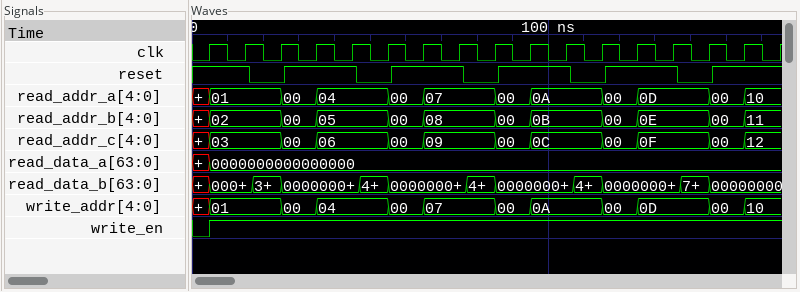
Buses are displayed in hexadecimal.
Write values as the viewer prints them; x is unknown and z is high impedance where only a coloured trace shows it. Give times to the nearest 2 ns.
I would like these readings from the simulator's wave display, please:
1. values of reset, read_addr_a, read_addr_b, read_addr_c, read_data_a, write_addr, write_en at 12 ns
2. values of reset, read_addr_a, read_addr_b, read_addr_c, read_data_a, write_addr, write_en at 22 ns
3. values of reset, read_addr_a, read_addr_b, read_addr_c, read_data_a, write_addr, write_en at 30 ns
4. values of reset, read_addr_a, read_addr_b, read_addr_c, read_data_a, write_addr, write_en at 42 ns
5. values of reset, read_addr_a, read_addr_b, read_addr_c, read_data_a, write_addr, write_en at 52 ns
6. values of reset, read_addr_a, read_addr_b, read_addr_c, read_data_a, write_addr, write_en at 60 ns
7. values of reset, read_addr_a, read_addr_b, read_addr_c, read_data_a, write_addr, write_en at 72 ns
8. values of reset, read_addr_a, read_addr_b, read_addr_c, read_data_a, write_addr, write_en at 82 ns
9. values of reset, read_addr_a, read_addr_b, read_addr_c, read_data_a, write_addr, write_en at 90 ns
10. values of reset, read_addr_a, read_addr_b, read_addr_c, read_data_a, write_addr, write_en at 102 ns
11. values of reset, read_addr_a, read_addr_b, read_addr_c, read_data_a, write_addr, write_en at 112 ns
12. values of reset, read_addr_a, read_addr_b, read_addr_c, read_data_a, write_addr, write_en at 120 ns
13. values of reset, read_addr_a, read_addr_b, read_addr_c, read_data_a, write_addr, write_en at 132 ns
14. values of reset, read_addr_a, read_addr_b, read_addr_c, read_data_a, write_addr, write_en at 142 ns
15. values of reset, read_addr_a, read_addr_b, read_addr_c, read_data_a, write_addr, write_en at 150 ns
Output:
reset=1, read_addr_a=01, read_addr_b=02, read_addr_c=03, read_data_a=0000000000000000, write_addr=01, write_en=1
reset=0, read_addr_a=01, read_addr_b=02, read_addr_c=03, read_data_a=0000000000000000, write_addr=01, write_en=1
reset=1, read_addr_a=00, read_addr_b=00, read_addr_c=00, read_data_a=0000000000000000, write_addr=00, write_en=1
reset=1, read_addr_a=04, read_addr_b=05, read_addr_c=06, read_data_a=0000000000000000, write_addr=04, write_en=1
reset=0, read_addr_a=04, read_addr_b=05, read_addr_c=06, read_data_a=0000000000000000, write_addr=04, write_en=1
reset=1, read_addr_a=00, read_addr_b=00, read_addr_c=00, read_data_a=0000000000000000, write_addr=00, write_en=1
reset=1, read_addr_a=07, read_addr_b=08, read_addr_c=09, read_data_a=0000000000000000, write_addr=07, write_en=1
reset=0, read_addr_a=07, read_addr_b=08, read_addr_c=09, read_data_a=0000000000000000, write_addr=07, write_en=1
reset=1, read_addr_a=00, read_addr_b=00, read_addr_c=00, read_data_a=0000000000000000, write_addr=00, write_en=1
reset=1, read_addr_a=0A, read_addr_b=0B, read_addr_c=0C, read_data_a=0000000000000000, write_addr=0A, write_en=1
reset=0, read_addr_a=0A, read_addr_b=0B, read_addr_c=0C, read_data_a=0000000000000000, write_addr=0A, write_en=1
reset=1, read_addr_a=00, read_addr_b=00, read_addr_c=00, read_data_a=0000000000000000, write_addr=00, write_en=1
reset=1, read_addr_a=0D, read_addr_b=0E, read_addr_c=0F, read_data_a=0000000000000000, write_addr=0D, write_en=1
reset=0, read_addr_a=0D, read_addr_b=0E, read_addr_c=0F, read_data_a=0000000000000000, write_addr=0D, write_en=1
reset=1, read_addr_a=00, read_addr_b=00, read_addr_c=00, read_data_a=0000000000000000, write_addr=00, write_en=1
